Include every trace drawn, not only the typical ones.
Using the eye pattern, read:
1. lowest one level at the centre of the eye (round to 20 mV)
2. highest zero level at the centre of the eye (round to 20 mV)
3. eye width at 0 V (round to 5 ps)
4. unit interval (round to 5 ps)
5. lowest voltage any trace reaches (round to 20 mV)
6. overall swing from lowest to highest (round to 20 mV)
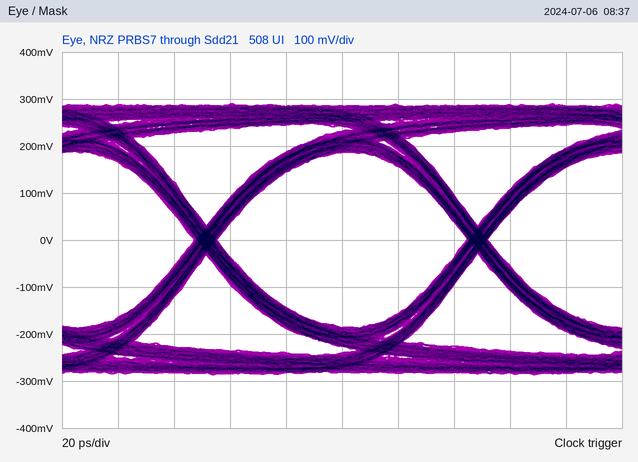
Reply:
180 mV
-180 mV
90 ps
95 ps
-280 mV
580 mV
